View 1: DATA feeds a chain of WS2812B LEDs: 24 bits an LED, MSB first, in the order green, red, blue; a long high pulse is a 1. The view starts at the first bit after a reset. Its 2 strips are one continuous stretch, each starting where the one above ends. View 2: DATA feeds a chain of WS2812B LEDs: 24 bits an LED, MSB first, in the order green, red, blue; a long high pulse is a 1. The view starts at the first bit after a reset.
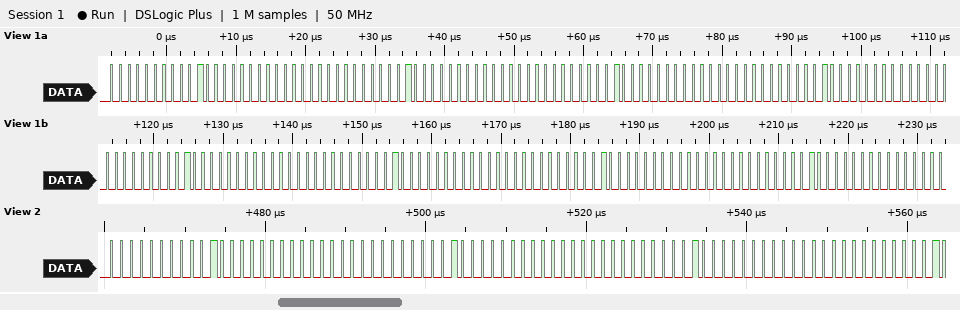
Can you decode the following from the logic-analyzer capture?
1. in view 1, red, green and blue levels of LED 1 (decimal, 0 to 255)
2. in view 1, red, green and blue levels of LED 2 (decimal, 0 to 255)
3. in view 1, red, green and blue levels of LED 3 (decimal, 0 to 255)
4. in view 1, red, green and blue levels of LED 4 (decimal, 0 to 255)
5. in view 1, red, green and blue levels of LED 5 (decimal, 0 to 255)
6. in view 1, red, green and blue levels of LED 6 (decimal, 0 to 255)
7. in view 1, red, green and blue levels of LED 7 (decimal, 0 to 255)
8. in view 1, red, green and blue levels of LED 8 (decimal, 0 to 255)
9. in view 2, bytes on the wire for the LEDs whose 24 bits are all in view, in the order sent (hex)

32, 0, 0
32, 0, 0
32, 0, 0
32, 0, 0
32, 0, 0
32, 0, 0
32, 0, 0
32, 0, 0
00 20 00 00 20 00 00 20 00
